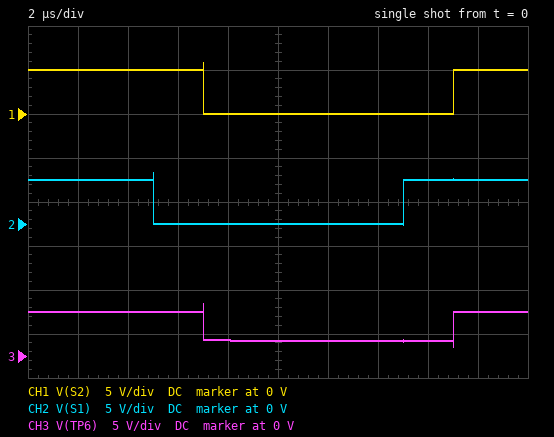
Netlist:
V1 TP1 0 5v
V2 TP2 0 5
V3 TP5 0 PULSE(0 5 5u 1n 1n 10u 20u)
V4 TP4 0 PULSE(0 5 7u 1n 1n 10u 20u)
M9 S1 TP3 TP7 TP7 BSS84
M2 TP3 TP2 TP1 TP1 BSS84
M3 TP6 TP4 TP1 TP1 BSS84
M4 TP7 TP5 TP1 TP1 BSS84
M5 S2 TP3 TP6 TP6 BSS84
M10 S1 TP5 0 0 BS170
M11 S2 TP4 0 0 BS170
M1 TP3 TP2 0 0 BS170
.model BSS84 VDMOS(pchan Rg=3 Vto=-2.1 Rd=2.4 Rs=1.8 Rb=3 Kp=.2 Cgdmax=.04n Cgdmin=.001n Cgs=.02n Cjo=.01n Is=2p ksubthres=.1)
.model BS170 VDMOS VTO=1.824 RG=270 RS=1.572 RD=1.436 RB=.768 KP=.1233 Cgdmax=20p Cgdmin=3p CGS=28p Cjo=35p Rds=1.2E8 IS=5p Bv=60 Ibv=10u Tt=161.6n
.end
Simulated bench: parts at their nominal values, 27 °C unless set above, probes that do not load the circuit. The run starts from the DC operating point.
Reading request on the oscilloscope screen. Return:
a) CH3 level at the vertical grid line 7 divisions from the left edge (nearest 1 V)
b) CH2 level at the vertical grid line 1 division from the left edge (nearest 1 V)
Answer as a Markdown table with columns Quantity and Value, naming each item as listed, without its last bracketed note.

| Quantity | Value |
|---|---|
| CH3 level at the vertical grid line 7 divisions from the left edge | 2 V |
| CH2 level at the vertical grid line 1 division from the left edge | 5 V |
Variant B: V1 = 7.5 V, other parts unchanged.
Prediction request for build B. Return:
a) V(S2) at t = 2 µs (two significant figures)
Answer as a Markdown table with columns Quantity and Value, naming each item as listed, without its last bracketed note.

| Quantity | Value |
|---|---|
| V(S2) at t = 2 µs | 7.5 V |
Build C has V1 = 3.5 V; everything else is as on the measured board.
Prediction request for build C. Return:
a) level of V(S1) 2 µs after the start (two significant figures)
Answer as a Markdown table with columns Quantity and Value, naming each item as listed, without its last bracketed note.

| Quantity | Value |
|---|---|
| level of V(S1) 2 µs after the start | 3.5 V |
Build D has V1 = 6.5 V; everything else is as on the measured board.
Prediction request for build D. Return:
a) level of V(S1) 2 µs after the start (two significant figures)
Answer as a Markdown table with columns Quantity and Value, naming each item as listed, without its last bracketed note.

| Quantity | Value |
|---|---|
| level of V(S1) 2 µs after the start | 6.5 V |
